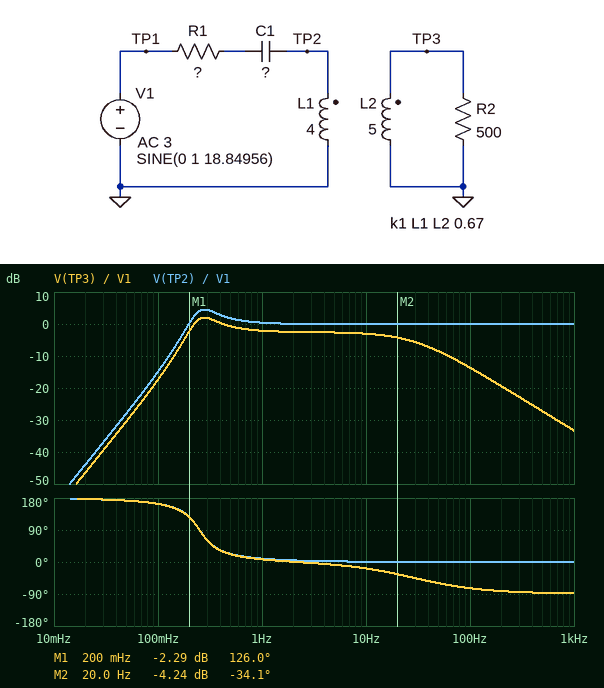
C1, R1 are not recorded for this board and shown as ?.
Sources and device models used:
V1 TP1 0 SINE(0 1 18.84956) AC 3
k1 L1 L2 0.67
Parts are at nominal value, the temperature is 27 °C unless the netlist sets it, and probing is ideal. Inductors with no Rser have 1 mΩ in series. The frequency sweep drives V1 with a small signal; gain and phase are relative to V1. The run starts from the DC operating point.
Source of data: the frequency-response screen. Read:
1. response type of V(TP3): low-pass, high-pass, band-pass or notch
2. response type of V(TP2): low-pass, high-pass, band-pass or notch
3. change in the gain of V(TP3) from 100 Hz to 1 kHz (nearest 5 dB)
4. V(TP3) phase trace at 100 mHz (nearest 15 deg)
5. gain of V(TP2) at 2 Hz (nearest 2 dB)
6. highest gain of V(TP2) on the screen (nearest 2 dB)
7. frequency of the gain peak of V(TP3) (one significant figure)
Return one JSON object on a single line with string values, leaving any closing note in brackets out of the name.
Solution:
{"response type of V(TP3): low-pass, high-pass, band-pass or notch": "band-pass", "response type of V(TP2): low-pass, high-pass, band-pass or notch": "high-pass", "change in the gain of V(TP3) from 100 Hz to 1 kHz": "-20 dB", "V(TP3) phase trace at 100 mHz": "165 deg", "gain of V(TP2) at 2 Hz": "0 dB", "highest gain of V(TP2) on the screen": "4 dB", "frequency of the gain peak of V(TP3)": "300 mHz"}
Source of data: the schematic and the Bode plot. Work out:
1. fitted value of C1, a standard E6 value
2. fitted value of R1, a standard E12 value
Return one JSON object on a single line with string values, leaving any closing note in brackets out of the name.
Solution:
{"fitted value of C1, a standard E6 value": "100 mF", "fitted value of R1, a standard E12 value": "3.9 Ω"}
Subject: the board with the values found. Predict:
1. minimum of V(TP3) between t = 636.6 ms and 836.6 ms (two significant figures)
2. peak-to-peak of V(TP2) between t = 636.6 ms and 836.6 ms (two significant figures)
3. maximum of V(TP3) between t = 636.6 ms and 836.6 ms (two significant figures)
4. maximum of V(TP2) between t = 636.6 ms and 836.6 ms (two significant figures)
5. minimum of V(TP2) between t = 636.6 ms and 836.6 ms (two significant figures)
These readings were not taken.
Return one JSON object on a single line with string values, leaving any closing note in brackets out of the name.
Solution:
{"minimum of V(TP3) between t = 636.6 ms and 836.6 ms": "-630 mV", "peak-to-peak of V(TP2) between t = 636.6 ms and 836.6 ms": "2.0 V", "maximum of V(TP3) between t = 636.6 ms and 836.6 ms": "620 mV", "maximum of V(TP2) between t = 636.6 ms and 836.6 ms": "990 mV", "minimum of V(TP2) between t = 636.6 ms and 836.6 ms": "-1.0 V"}
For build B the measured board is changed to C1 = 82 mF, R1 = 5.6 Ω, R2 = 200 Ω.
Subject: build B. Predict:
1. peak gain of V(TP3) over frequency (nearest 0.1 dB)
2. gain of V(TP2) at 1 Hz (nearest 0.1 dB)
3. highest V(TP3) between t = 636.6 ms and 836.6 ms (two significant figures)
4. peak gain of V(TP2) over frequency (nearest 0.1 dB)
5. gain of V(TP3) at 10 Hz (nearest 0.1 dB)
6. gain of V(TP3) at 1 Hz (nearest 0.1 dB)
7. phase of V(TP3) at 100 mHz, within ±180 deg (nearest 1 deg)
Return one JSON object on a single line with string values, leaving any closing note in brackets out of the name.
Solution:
{"peak gain of V(TP3) over frequency": "-0.1 dB", "gain of V(TP2) at 1 Hz": "0.3 dB", "highest V(TP3) between t = 636.6 ms and 836.6 ms": "380 mV", "peak gain of V(TP2) over frequency": "2.4 dB", "gain of V(TP3) at 10 Hz": "-5.0 dB", "gain of V(TP3) at 1 Hz": "-2.2 dB", "phase of V(TP3) at 100 mHz, within ±180 deg": "161 deg"}
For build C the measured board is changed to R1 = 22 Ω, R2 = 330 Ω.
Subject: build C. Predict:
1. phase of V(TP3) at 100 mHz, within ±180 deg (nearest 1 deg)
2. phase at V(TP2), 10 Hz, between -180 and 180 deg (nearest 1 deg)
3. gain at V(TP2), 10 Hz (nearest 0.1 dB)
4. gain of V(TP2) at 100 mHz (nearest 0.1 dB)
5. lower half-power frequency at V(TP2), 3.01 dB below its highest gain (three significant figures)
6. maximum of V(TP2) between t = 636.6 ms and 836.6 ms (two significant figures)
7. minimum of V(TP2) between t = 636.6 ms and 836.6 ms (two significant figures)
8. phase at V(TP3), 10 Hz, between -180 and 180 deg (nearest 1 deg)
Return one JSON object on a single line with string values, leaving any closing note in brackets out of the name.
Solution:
{"phase of V(TP3) at 100 mHz, within ±180 deg": "121 deg", "phase at V(TP2), 10 Hz, between -180 and 180 deg": "6 deg", "gain at V(TP2), 10 Hz": "-0.3 dB", "gain of V(TP2) at 100 mHz": "-20.2 dB", "lower half-power frequency at V(TP2), 3.01 dB below its highest gain": "837 mHz", "maximum of V(TP2) between t = 636.6 ms and 836.6 ms": "980 mV", "minimum of V(TP2) between t = 636.6 ms and 836.6 ms": "-980 mV", "phase at V(TP3), 10 Hz, between -180 and 180 deg": "-22 deg"}
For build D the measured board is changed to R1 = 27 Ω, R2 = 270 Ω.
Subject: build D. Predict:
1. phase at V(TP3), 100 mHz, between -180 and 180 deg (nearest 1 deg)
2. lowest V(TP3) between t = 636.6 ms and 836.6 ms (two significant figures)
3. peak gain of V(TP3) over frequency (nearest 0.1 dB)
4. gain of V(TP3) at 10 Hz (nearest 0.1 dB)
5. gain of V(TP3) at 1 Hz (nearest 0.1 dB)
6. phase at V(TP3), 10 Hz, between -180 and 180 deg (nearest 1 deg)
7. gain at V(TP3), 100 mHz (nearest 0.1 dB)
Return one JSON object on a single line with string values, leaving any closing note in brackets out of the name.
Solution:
{"phase at V(TP3), 100 mHz, between -180 and 180 deg": "116 deg", "lowest V(TP3) between t = 636.6 ms and 836.6 ms": "-470 mV", "peak gain of V(TP3) over frequency": "-3.5 dB", "gain of V(TP3) at 10 Hz": "-4.4 dB", "gain of V(TP3) at 1 Hz": "-5.9 dB", "phase at V(TP3), 10 Hz, between -180 and 180 deg": "-25 deg", "gain at V(TP3), 100 mHz": "-24.1 dB"}
